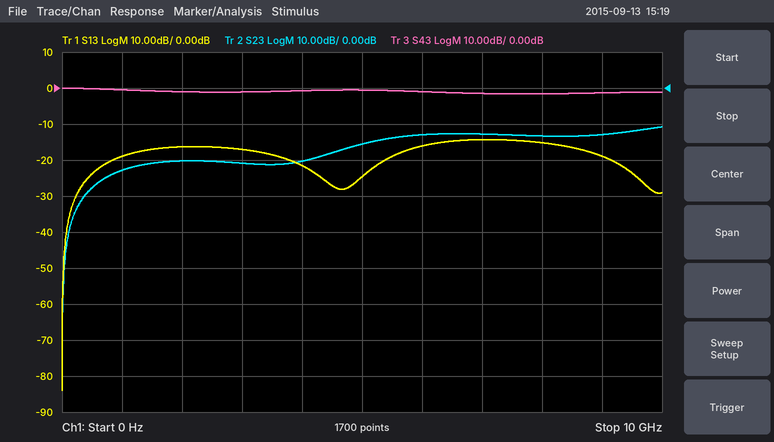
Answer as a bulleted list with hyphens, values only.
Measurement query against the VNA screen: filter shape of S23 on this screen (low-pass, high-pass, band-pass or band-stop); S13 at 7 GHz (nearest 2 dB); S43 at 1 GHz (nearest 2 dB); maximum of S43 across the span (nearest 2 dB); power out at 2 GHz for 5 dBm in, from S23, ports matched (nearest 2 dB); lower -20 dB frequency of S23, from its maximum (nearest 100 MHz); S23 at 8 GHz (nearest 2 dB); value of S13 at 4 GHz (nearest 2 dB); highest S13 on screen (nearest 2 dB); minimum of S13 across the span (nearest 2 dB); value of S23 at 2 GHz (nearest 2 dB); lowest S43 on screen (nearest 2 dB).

- high-pass
- -14 dB
- 0 dB
- 0 dB
- -16 dBm
- 300 MHz
- -14 dB
- -22 dB
- -14 dB
- -84 dB
- -20 dB
- -2 dB
